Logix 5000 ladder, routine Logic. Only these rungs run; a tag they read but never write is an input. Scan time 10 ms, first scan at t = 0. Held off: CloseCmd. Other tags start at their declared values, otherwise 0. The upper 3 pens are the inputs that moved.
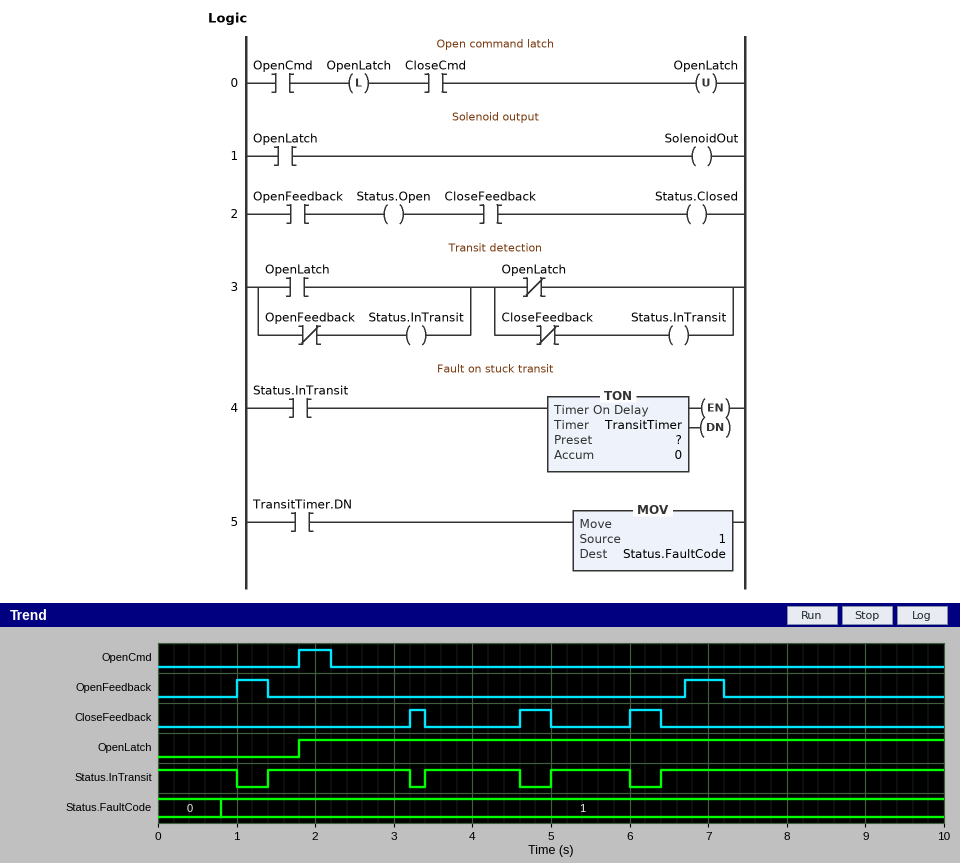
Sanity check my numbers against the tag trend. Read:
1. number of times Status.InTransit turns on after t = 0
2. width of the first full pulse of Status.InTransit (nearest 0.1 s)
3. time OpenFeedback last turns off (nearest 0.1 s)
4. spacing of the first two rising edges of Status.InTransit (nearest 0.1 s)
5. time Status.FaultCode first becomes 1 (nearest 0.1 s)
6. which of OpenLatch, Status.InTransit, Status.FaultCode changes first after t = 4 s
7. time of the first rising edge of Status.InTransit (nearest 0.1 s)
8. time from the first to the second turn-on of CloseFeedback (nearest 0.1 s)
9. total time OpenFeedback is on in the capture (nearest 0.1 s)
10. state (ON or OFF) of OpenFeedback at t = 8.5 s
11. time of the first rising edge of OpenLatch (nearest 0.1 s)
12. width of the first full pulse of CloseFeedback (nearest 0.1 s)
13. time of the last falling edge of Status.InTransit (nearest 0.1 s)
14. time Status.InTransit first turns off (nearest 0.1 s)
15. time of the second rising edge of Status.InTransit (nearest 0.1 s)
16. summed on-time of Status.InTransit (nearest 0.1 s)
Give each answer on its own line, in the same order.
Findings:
4
1.8 s
7.2 s
2.0 s
0.8 s
Status.InTransit
1.4 s
1.4 s
0.9 s
OFF
1.8 s
0.2 s
6.0 s
1.0 s
3.4 s
8.6 s
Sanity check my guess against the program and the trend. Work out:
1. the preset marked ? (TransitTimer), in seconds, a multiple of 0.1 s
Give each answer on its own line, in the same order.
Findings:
0.8 s
